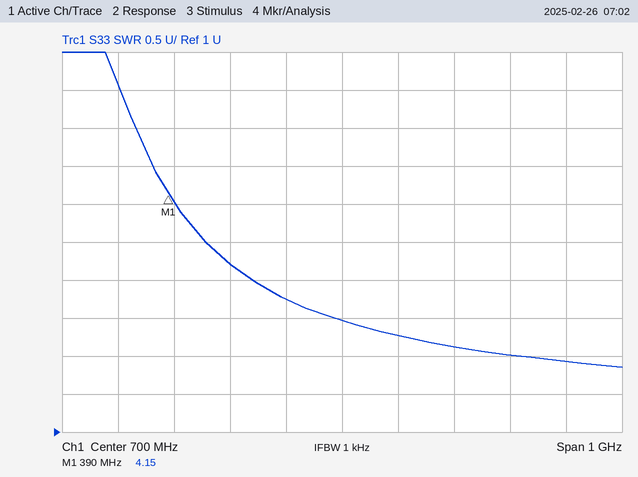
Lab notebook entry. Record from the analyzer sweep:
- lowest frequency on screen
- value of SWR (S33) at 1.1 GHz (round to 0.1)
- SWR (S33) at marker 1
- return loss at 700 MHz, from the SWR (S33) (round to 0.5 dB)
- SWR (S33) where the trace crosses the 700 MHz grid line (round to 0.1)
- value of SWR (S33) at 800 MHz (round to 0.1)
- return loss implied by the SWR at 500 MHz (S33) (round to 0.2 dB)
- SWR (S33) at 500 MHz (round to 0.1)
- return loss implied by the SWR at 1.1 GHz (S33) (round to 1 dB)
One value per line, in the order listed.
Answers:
200 MHz
1.9
4.15
7.5 dB
2.5
2.3
5.6 dB
3.2
10 dB
